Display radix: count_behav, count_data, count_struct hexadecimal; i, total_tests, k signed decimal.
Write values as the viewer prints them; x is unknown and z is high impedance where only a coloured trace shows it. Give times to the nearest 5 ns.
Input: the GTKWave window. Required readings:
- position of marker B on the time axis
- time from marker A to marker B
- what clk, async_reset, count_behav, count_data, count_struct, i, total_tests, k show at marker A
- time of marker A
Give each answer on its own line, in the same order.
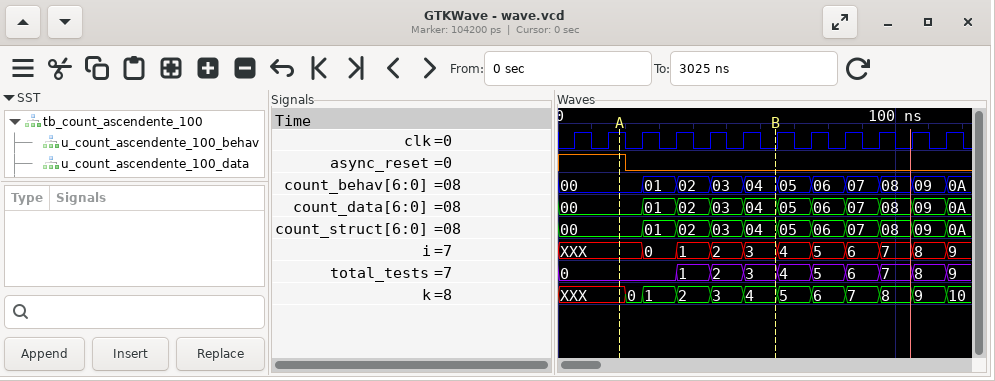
65 ns
45 ns
clk=1, async_reset=1, count_behav=00, count_data=00, count_struct=00, i=XXX, total_tests=0, k=XXX
20 ns
